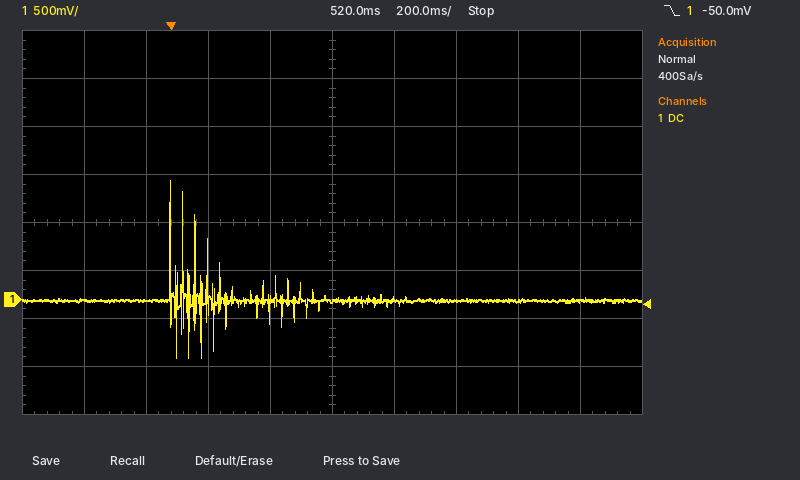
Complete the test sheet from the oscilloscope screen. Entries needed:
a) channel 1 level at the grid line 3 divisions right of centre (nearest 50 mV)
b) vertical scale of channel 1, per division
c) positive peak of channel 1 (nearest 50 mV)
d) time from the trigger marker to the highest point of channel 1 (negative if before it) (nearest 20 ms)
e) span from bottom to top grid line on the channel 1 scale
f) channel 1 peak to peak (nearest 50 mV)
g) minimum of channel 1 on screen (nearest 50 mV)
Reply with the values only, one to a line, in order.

0 mV
500 mV
1.25 V
0 ms
4 V
1.85 V
-600 mV
